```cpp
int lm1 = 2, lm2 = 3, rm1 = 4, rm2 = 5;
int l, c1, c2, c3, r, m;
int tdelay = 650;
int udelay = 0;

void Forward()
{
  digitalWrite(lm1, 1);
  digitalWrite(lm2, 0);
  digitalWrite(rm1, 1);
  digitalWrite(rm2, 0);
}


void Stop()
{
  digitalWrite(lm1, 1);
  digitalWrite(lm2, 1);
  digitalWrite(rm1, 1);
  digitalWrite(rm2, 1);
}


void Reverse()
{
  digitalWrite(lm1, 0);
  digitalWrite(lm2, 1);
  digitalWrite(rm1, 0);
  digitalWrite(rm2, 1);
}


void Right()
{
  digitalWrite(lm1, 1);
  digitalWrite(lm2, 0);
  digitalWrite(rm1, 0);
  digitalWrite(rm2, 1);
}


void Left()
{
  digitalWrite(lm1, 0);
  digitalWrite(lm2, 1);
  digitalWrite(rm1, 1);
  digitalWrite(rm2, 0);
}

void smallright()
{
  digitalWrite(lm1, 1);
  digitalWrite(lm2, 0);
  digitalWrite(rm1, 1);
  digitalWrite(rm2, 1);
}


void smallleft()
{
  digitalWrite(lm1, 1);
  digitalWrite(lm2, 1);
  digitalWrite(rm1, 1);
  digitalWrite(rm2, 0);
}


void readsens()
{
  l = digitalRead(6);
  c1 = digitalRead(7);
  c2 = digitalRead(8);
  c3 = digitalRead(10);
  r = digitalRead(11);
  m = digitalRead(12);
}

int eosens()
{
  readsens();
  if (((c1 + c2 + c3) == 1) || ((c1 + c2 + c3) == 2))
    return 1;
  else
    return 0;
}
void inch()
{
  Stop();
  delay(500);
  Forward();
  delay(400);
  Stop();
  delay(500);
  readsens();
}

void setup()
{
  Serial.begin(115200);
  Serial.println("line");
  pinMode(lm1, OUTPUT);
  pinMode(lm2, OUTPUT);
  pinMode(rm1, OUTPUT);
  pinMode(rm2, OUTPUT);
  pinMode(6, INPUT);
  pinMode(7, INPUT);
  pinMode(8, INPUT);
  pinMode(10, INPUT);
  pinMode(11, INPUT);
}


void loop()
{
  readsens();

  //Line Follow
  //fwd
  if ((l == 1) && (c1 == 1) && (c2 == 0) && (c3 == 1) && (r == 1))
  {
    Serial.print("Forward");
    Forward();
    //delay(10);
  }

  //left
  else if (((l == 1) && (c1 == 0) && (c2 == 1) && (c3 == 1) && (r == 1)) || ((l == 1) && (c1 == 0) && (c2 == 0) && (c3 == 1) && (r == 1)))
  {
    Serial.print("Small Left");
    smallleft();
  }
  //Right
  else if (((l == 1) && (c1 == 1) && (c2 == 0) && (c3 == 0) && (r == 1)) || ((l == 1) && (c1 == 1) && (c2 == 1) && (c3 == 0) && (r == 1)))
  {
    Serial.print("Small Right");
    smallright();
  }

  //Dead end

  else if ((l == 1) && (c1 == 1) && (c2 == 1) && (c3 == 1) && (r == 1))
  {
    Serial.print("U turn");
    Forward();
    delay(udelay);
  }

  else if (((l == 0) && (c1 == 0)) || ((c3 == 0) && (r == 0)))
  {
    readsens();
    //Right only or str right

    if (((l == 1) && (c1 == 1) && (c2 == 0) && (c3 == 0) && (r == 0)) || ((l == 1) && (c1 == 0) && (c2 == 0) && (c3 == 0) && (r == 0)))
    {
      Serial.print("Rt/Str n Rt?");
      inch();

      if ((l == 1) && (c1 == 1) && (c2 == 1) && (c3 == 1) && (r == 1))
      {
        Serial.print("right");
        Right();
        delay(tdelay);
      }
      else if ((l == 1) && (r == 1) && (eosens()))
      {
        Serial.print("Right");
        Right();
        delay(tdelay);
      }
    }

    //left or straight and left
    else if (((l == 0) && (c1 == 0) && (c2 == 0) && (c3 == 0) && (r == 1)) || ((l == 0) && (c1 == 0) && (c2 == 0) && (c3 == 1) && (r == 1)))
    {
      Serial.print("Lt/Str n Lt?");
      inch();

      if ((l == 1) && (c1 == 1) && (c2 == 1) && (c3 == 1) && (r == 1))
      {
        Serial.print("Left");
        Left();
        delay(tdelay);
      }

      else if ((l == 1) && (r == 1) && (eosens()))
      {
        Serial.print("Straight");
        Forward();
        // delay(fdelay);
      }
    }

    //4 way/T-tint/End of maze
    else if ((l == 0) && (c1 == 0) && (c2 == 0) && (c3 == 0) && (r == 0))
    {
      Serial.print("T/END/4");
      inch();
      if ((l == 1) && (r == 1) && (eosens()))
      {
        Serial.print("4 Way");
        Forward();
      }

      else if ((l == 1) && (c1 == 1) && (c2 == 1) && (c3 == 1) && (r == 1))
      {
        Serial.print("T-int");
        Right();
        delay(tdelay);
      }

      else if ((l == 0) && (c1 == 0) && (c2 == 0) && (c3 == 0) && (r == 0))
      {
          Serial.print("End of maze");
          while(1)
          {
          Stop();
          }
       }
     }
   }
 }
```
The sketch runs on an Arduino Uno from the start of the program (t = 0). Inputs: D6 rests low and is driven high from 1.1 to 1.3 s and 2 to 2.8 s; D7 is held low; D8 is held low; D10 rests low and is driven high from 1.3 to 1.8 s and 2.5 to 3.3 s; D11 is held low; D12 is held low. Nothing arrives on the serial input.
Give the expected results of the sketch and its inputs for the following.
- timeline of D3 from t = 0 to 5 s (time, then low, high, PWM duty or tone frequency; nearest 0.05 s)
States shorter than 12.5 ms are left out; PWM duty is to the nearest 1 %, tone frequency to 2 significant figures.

0 s high; 0.5 s low; 0.9 s high; 2.3 s low; 2.7 s high; 3.8 s low; 4.2 s high
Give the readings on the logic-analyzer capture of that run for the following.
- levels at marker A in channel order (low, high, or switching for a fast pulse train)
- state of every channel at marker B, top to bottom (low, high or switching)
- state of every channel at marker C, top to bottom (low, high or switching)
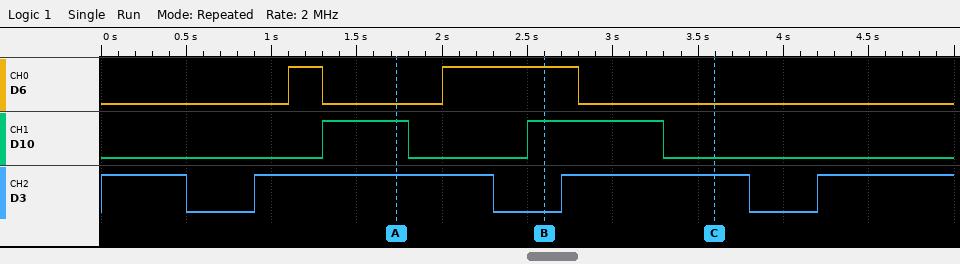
D6 low, D10 high, D3 high
D6 high, D10 high, D3 low
D6 low, D10 low, D3 high
